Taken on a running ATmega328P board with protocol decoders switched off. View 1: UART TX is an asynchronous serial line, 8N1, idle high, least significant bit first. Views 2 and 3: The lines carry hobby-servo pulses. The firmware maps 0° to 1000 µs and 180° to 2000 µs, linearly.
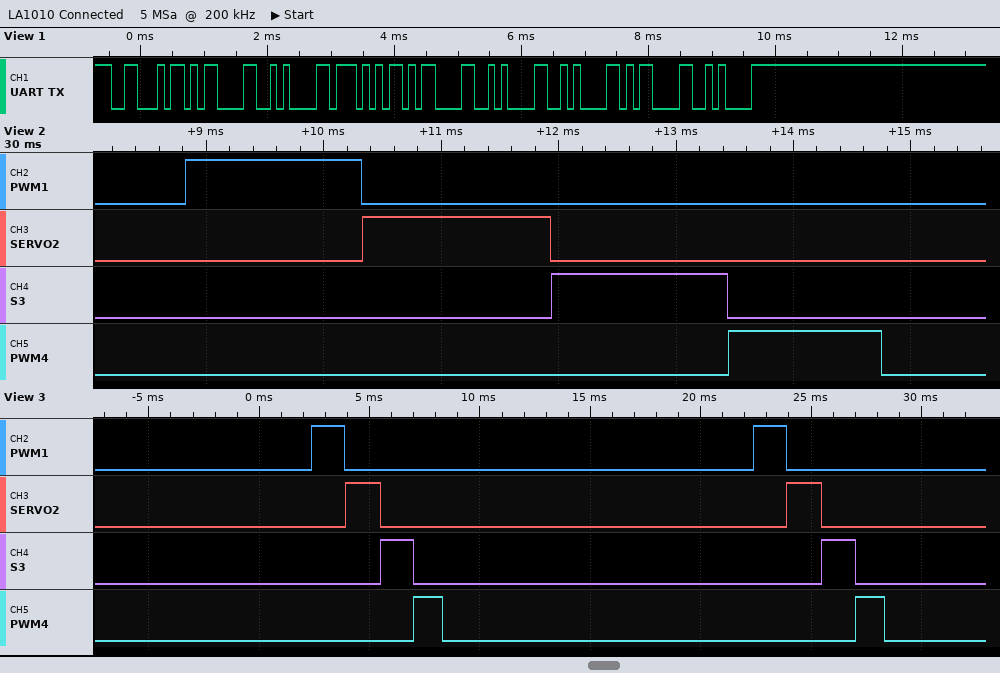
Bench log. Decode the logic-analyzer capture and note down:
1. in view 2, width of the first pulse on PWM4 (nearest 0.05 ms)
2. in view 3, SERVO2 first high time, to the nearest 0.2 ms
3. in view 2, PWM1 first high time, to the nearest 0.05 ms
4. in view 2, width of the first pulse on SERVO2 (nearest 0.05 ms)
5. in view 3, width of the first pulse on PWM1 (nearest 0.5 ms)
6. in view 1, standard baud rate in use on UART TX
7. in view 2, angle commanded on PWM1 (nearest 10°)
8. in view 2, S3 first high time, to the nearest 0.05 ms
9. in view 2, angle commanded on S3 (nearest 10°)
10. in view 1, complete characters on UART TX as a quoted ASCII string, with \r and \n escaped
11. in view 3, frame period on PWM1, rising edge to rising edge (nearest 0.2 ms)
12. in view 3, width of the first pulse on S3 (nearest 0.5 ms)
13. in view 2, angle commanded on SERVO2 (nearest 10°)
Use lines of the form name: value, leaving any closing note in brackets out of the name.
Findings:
in view 2, width of the first pulse on PWM4: 1.30 ms
in view 3, SERVO2 first high time, to the nearest 0.2 ms: 1.6 ms
in view 2, PWM1 first high time, to the nearest 0.05 ms: 1.50 ms
in view 2, width of the first pulse on SERVO2: 1.60 ms
in view 3, width of the first pulse on PWM1: 1.5 ms
in view 1, standard baud rate in use on UART TX: 9600 baud
in view 2, angle commanded on PWM1: 90°
in view 2, S3 first high time, to the nearest 0.05 ms: 1.50 ms
in view 2, angle commanded on S3: 90°
in view 1, complete characters on UART TX as a quoted ASCII string, with \r and \n escaped: "F\r\nW\r\n\n\r\n"
in view 3, frame period on PWM1, rising edge to rising edge: 20.0 ms
in view 3, width of the first pulse on S3: 1.5 ms
in view 2, angle commanded on SERVO2: 110°
